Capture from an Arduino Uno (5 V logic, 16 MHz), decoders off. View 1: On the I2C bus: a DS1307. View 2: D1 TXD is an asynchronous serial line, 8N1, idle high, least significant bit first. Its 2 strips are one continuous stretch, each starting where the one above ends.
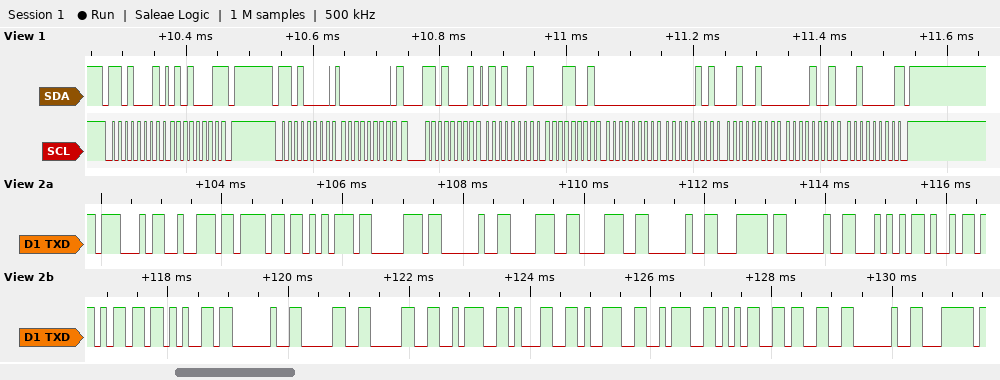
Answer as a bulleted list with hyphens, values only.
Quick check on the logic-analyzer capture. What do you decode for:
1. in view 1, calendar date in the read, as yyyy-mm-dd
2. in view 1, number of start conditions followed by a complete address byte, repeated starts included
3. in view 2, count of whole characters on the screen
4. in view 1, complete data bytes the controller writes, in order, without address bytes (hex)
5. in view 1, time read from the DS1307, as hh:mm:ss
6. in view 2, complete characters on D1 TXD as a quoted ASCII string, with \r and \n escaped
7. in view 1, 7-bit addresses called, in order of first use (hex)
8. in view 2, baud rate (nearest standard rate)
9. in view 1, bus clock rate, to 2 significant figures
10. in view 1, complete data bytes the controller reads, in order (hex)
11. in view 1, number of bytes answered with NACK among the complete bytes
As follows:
- 2020-09-24
- 3
- 26
- 00
- 00:19:51
- "Group 88 | Time 00:19:53 |"
- 0x68
- 9600 baud
- 100 kHz
- 51 51 19 00 05 24 09 20
- 2
